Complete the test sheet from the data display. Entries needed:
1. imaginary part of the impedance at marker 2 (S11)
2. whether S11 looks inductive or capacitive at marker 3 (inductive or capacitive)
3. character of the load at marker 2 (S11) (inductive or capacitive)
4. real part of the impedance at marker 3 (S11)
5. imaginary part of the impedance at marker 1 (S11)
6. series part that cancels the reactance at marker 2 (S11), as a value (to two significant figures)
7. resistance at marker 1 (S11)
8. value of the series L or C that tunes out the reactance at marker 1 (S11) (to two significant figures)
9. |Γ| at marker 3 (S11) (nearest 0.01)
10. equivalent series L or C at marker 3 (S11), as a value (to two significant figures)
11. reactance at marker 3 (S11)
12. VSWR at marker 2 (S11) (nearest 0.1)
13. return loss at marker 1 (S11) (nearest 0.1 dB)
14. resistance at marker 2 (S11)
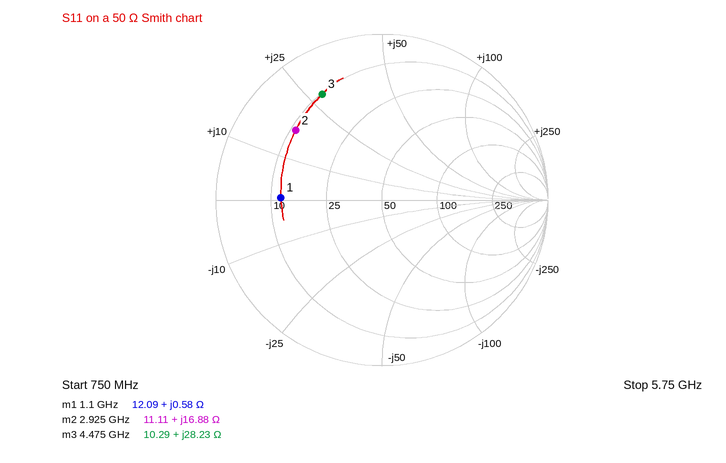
+16.88 Ω
inductive
inductive
10.29 Ω
+0.58 Ω
3.2 pF
12.09 Ω
250 pF
0.73
1.0 nH
+28.23 Ω
5.0
4.3 dB
11.11 Ω
